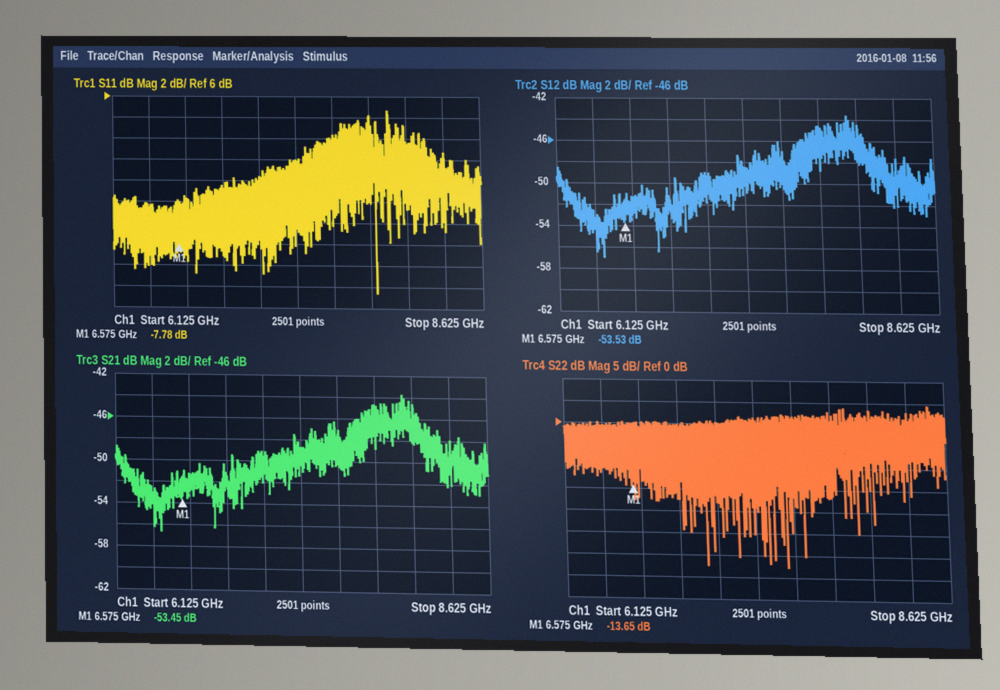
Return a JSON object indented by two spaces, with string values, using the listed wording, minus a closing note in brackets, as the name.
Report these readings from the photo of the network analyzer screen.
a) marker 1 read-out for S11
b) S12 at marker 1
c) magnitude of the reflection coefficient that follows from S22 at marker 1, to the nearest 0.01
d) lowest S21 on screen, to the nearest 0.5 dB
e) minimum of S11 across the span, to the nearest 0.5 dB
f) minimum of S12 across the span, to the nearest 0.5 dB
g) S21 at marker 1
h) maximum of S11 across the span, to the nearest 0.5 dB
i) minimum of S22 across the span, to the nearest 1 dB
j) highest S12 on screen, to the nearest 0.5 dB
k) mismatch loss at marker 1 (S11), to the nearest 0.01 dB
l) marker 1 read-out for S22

{
  "marker 1 read-out for S11": "-7.78 dB",
  "S12 at marker 1": "-53.53 dB",
  "magnitude of the reflection coefficient that follows from S22 at marker 1, to the nearest 0.01": "0.21",
  "lowest S21 on screen, to the nearest 0.5 dB": "-56.5 dB",
  "minimum of S11 across the span, to the nearest 0.5 dB": "-12.5 dB",
  "minimum of S12 across the span, to the nearest 0.5 dB": "-57.0 dB",
  "S21 at marker 1": "-53.45 dB",
  "maximum of S11 across the span, to the nearest 0.5 dB": "4.5 dB",
  "minimum of S22 across the span, to the nearest 1 dB": "-33 dB",
  "highest S12 on screen, to the nearest 0.5 dB": "-43.5 dB",
  "mismatch loss at marker 1 (S11), to the nearest 0.01 dB": "0.79 dB",
  "marker 1 read-out for S22": "-13.65 dB"
}
